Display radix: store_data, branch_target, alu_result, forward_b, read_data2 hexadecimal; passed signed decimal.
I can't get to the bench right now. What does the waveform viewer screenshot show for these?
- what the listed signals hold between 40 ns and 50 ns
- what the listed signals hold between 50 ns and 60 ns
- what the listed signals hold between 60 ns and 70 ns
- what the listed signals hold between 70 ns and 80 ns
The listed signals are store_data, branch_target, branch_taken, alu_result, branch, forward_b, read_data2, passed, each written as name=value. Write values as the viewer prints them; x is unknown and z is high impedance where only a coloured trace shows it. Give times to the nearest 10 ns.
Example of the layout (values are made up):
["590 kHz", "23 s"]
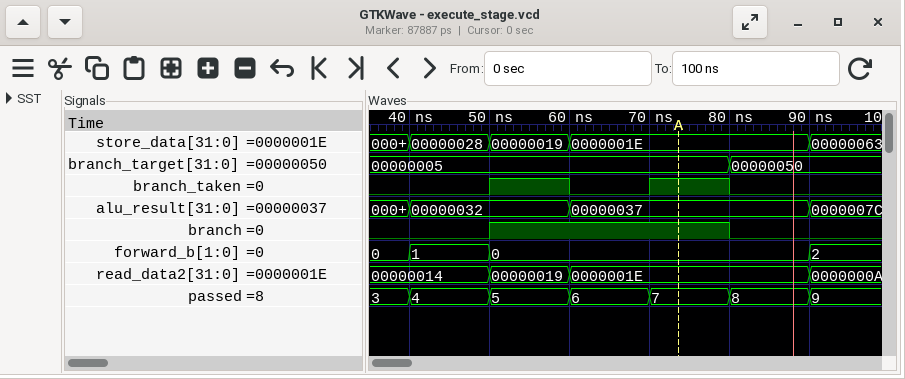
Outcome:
["store_data=00000028, branch_target=00000005, branch_taken=0, alu_result=00000032, branch=0, forward_b=1, read_data2=00000014, passed=4", "store_data=00000019, branch_target=00000005, branch_taken=1, alu_result=00000032, branch=1, forward_b=0, read_data2=00000019, passed=5", "store_data=0000001E, branch_target=00000005, branch_taken=0, alu_result=00000037, branch=1, forward_b=0, read_data2=0000001E, passed=6", "store_data=0000001E, branch_target=00000005, branch_taken=1, alu_result=00000037, branch=1, forward_b=0, read_data2=0000001E, passed=7"]
